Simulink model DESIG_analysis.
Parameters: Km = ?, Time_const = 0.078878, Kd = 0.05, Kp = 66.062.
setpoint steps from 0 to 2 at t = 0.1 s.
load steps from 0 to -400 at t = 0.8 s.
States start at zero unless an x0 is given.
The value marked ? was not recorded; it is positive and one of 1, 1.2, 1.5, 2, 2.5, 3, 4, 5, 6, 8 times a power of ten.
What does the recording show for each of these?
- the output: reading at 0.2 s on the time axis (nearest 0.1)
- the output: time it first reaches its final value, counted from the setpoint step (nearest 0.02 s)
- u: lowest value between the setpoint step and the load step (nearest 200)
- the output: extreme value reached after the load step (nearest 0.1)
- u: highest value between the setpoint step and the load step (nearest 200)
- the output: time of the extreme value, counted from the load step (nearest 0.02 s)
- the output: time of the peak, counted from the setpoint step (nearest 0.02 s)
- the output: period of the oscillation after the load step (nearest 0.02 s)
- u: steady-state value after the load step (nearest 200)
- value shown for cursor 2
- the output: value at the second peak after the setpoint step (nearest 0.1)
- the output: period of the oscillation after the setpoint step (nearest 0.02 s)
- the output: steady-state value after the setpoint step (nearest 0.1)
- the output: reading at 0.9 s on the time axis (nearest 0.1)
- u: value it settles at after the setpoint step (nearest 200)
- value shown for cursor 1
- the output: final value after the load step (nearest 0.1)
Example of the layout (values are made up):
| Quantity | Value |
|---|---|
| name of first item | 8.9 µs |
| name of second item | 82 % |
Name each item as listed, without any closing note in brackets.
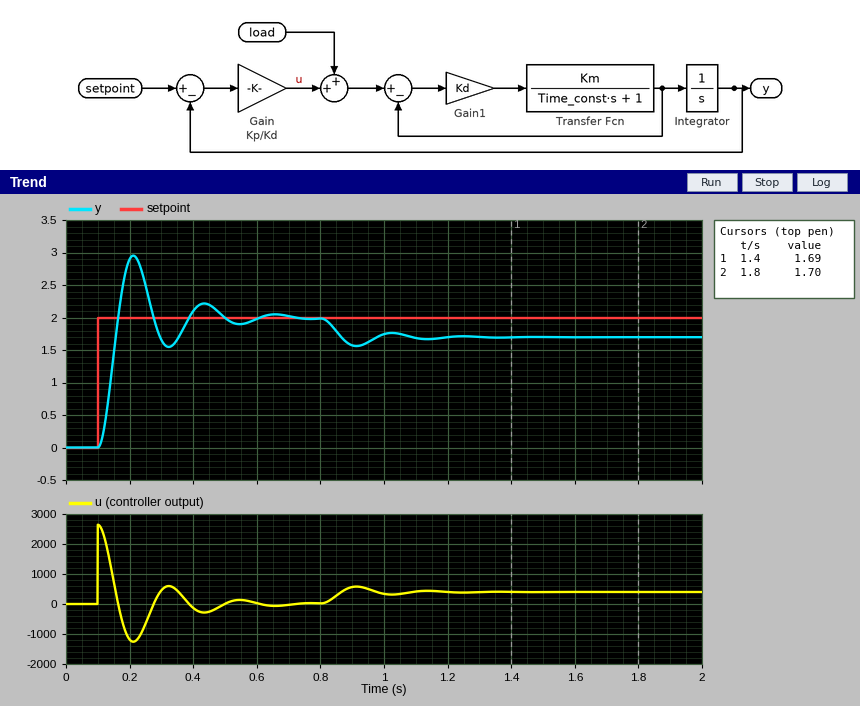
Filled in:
| Quantity | Value |
|---|---|
| the output: reading at 0.2 s on the time axis | 2.9 |
| the output: time it first reaches its final value, counted from the setpoint step | 0.06 s |
| u: lowest value between the setpoint step and the load step | -1200 |
| the output: extreme value reached after the load step | 1.6 |
| u: highest value between the setpoint step and the load step | 2600 |
| the output: time of the extreme value, counted from the load step | 0.12 s |
| the output: time of the peak, counted from the setpoint step | 0.12 s |
| the output: period of the oscillation after the load step | 0.22 s |
| u: steady-state value after the load step | 400 |
| value shown for cursor 2 | 1.70 |
| the output: value at the second peak after the setpoint step | 2.2 |
| the output: period of the oscillation after the setpoint step | 0.22 s |
| the output: steady-state value after the setpoint step | 2.0 |
| the output: reading at 0.9 s on the time axis | 1.6 |
| u: value it settles at after the setpoint step | 0 |
| value shown for cursor 1 | 1.69 |
| the output: final value after the load step | 1.7 |
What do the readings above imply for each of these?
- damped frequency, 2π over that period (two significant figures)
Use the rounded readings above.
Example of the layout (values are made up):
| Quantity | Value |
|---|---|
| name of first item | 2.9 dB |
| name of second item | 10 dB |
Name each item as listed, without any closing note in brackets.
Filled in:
| Quantity | Value |
|---|---|
| damped frequency, 2π over that period | 29 rad/s |
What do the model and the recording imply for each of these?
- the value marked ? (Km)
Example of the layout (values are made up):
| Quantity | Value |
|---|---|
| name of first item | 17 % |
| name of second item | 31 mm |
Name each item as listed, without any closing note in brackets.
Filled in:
| Quantity | Value |
|---|---|
| the value marked ? | 1 |
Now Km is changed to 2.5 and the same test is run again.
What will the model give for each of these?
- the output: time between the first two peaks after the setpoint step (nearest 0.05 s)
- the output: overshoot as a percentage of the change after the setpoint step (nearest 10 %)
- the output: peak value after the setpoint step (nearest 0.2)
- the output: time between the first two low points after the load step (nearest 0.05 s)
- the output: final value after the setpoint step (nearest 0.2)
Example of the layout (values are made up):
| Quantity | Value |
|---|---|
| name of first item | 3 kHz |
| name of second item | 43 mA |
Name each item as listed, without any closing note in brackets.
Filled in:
| Quantity | Value |
|---|---|
| the output: time between the first two peaks after the setpoint step | 0.15 s |
| the output: overshoot as a percentage of the change after the setpoint step | 60 % |
| the output: peak value after the setpoint step | 3.2 |
| the output: time between the first two low points after the load step | 0.15 s |
| the output: final value after the setpoint step | 2.0 |
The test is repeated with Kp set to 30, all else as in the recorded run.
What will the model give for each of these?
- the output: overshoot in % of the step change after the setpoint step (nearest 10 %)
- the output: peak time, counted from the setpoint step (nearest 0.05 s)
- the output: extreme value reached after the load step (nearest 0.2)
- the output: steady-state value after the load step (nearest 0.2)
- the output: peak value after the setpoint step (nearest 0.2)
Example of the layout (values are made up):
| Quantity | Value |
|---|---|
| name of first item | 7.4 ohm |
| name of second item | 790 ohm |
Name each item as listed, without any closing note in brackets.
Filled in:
| Quantity | Value |
|---|---|
| the output: overshoot in % of the step change after the setpoint step | 30 % |
| the output: peak time, counted from the setpoint step | 0.15 s |
| the output: extreme value reached after the load step | 1.2 |
| the output: steady-state value after the load step | 1.4 |
| the output: peak value after the setpoint step | 2.6 |
